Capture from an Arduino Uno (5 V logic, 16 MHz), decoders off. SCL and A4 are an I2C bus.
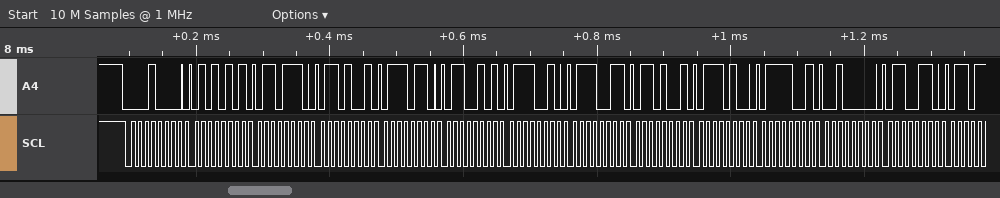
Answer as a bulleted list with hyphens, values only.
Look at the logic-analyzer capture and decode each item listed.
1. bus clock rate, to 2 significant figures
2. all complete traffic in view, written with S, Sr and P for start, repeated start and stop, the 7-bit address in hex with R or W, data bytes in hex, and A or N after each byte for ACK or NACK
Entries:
- 100 kHz
- S 08W A 55 A 6E A 69 A 76 A 65 A 72 A 73 A 69 A 74 A 79 A 20 A 66 A
